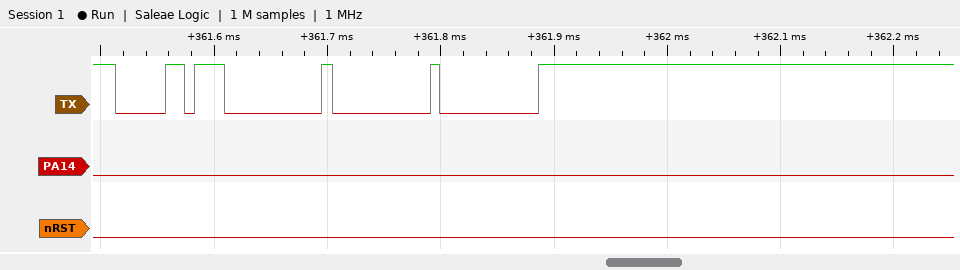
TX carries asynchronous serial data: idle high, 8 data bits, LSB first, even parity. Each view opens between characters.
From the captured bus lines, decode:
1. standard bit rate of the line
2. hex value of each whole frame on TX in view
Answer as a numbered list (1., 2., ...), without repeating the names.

1. 115200 baud
2. B0, 00, 00, 00
